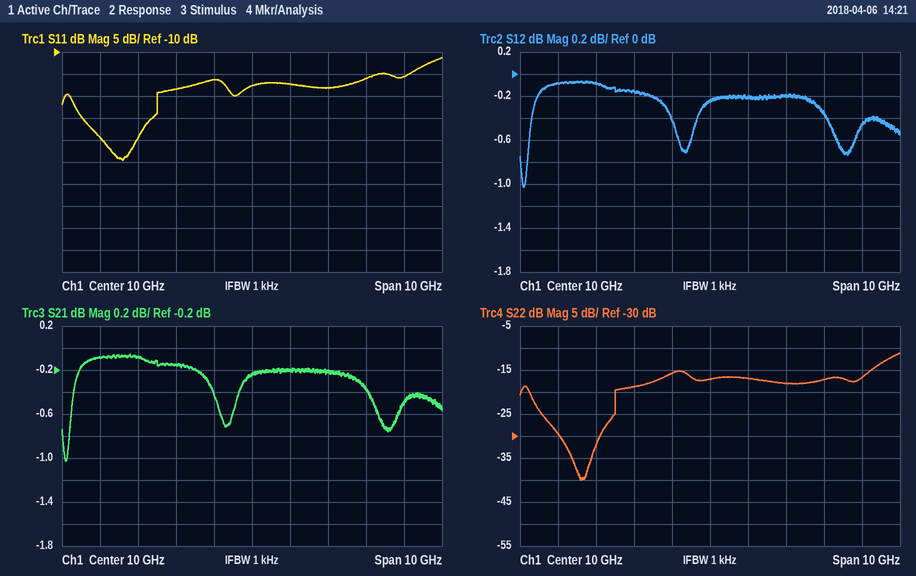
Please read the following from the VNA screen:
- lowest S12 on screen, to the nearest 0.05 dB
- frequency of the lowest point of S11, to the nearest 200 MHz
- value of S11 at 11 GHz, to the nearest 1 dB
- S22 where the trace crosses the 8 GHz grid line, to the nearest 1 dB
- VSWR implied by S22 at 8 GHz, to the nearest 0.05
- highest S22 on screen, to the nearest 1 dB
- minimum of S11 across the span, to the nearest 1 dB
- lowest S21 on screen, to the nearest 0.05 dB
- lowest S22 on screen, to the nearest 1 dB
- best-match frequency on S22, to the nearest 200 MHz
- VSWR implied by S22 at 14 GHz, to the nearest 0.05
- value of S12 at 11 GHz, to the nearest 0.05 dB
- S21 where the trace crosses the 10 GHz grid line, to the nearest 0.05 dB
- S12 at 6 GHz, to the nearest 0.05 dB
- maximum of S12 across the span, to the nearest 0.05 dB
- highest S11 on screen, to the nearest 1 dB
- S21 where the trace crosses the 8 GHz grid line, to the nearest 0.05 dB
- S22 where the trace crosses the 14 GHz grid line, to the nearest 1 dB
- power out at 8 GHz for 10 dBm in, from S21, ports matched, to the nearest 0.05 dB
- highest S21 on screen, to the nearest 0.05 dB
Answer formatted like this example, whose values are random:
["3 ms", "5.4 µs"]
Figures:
["-1.05 dB", "6.6 GHz", "-17 dB", "-19 dB", "1.25", "-11 dB", "-35 dB", "-1.05 dB", "-40 dB", "6.6 GHz", "1.35", "-0.20 dB", "-0.25 dB", "-0.10 dB", "-0.05 dB", "-11 dB", "-0.15 dB", "-17 dB", "9.85 dBm", "-0.05 dB"]
